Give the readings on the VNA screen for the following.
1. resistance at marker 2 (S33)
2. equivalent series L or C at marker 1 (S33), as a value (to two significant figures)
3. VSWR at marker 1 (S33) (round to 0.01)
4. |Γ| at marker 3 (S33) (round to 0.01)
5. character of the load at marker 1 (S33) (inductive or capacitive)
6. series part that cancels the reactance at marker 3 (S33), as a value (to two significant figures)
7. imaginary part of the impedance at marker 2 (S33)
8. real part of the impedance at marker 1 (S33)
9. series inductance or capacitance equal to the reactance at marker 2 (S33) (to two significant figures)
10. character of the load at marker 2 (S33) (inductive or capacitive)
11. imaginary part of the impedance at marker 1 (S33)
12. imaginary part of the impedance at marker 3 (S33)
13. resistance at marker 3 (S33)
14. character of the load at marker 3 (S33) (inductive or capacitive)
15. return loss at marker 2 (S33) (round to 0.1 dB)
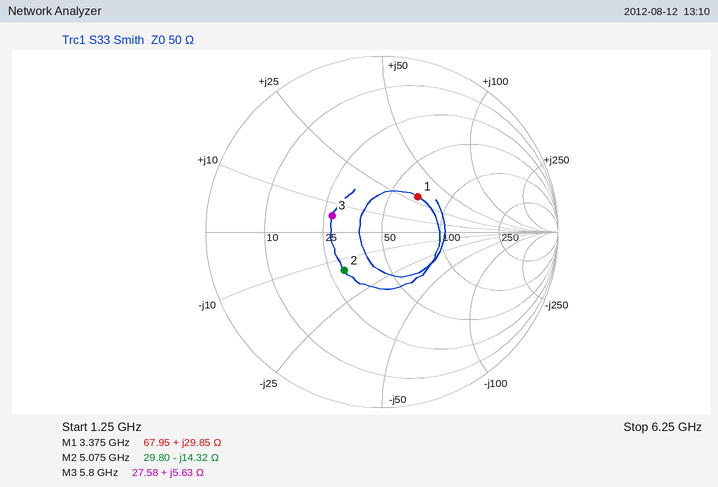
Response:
29.80 Ω
1.4 nH
1.80
0.30
inductive
4.9 pF
-14.32 Ω
67.95 Ω
2.2 pF
capacitive
+29.85 Ω
+5.63 Ω
27.58 Ω
inductive
10.3 dB
